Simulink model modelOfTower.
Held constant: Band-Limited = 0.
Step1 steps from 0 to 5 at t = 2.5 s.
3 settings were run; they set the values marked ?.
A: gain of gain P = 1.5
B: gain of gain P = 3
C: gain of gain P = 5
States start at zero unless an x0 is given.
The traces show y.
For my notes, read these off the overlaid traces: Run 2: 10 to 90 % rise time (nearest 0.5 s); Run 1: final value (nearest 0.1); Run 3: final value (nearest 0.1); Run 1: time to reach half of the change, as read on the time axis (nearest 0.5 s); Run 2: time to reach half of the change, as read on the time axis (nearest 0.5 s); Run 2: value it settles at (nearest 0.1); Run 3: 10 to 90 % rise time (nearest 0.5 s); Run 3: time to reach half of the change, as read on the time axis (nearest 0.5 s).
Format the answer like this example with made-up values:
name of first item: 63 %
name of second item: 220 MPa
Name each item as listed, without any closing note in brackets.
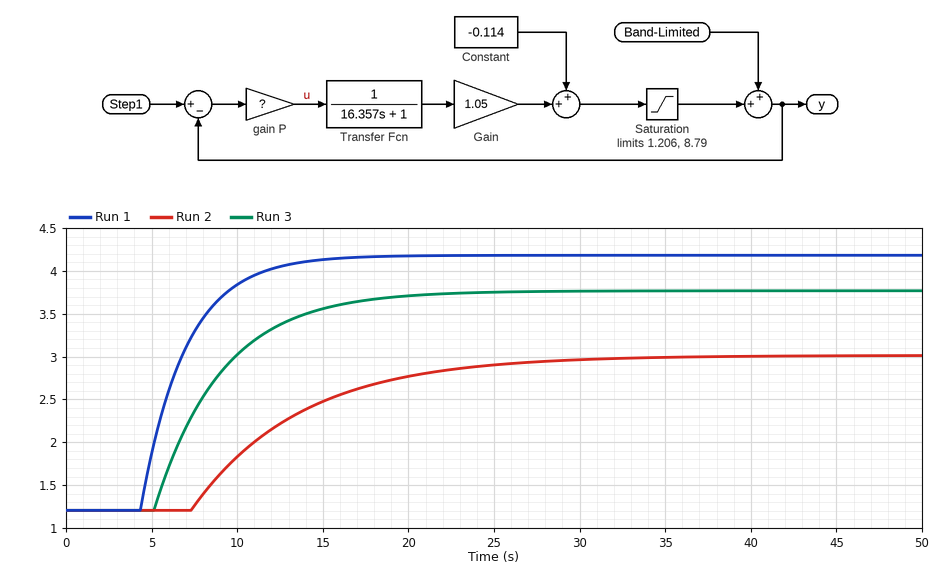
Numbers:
Run 2: 10 to 90 % rise time: 14.0 s
Run 1: final value: 4.2
Run 3: final value: 3.8
Run 1: time to reach half of the change, as read on the time axis: 6.0 s
Run 2: time to reach half of the change, as read on the time axis: 11.5 s
Run 2: value it settles at: 3.0
Run 3: 10 to 90 % rise time: 8.5 s
Run 3: time to reach half of the change, as read on the time axis: 8.0 s
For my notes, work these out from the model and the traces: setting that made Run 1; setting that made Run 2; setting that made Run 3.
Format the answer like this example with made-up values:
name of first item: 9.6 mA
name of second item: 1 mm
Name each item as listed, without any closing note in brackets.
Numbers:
setting that made Run 1: C
setting that made Run 2: A
setting that made Run 3: B
